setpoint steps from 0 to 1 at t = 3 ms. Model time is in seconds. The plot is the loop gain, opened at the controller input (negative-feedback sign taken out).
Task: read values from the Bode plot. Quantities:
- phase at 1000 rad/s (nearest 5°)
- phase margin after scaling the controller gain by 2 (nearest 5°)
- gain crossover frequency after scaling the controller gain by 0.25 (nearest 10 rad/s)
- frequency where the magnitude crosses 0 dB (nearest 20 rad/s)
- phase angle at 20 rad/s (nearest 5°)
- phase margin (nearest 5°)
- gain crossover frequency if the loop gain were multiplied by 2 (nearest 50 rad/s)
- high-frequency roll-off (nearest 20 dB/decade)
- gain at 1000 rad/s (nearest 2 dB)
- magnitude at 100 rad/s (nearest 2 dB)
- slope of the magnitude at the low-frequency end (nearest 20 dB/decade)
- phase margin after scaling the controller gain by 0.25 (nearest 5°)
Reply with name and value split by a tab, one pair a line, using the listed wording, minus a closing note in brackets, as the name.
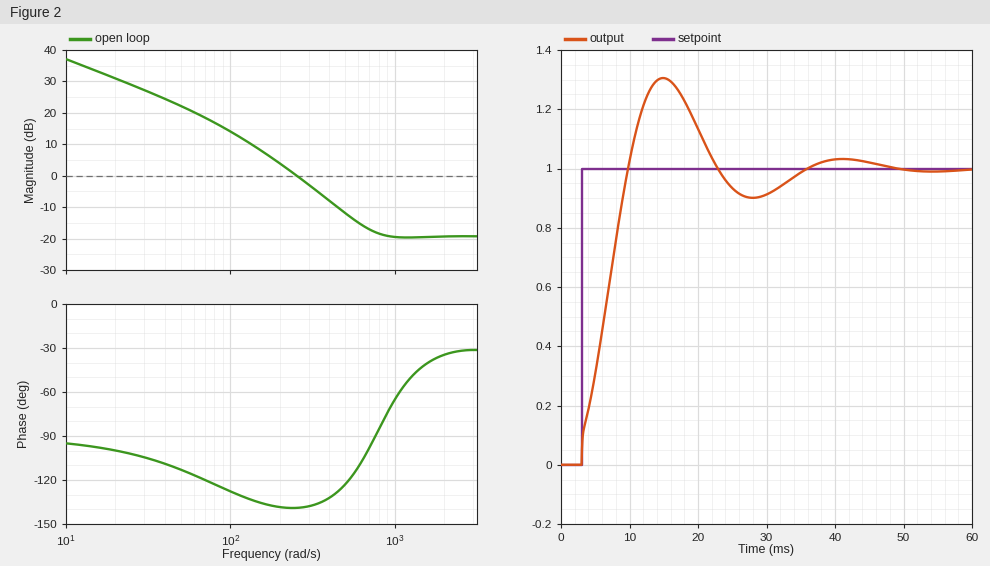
phase at 1000 rad/s	-65°
phase margin after scaling the controller gain by 2	45°
gain crossover frequency after scaling the controller gain by 0.25	120 rad/s
frequency where the magnitude crosses 0 dB	260 rad/s
phase angle at 20 rad/s	-100°
phase margin	40°
gain crossover frequency if the loop gain were multiplied by 2	350 rad/s
high-frequency roll-off	0 dB/decade
gain at 1000 rad/s	-20 dB
magnitude at 100 rad/s	14 dB
slope of the magnitude at the low-frequency end	-20 dB/decade
phase margin after scaling the controller gain by 0.25	50°
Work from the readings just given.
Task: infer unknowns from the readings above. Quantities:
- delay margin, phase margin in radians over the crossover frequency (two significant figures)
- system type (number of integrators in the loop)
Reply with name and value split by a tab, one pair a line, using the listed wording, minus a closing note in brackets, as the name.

delay margin, phase margin in radians over the crossover frequency	0.0027 s
system type	1
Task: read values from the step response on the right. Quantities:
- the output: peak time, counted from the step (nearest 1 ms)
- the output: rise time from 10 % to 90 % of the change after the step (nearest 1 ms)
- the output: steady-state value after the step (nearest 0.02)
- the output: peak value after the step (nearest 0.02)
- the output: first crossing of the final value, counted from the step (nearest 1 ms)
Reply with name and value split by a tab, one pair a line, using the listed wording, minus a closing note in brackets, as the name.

the output: peak time, counted from the step	12 ms
the output: rise time from 10 % to 90 % of the change after the step	6 ms
the output: steady-state value after the step	1.00
the output: peak value after the step	1.30
the output: first crossing of the final value, counted from the step	7 ms
